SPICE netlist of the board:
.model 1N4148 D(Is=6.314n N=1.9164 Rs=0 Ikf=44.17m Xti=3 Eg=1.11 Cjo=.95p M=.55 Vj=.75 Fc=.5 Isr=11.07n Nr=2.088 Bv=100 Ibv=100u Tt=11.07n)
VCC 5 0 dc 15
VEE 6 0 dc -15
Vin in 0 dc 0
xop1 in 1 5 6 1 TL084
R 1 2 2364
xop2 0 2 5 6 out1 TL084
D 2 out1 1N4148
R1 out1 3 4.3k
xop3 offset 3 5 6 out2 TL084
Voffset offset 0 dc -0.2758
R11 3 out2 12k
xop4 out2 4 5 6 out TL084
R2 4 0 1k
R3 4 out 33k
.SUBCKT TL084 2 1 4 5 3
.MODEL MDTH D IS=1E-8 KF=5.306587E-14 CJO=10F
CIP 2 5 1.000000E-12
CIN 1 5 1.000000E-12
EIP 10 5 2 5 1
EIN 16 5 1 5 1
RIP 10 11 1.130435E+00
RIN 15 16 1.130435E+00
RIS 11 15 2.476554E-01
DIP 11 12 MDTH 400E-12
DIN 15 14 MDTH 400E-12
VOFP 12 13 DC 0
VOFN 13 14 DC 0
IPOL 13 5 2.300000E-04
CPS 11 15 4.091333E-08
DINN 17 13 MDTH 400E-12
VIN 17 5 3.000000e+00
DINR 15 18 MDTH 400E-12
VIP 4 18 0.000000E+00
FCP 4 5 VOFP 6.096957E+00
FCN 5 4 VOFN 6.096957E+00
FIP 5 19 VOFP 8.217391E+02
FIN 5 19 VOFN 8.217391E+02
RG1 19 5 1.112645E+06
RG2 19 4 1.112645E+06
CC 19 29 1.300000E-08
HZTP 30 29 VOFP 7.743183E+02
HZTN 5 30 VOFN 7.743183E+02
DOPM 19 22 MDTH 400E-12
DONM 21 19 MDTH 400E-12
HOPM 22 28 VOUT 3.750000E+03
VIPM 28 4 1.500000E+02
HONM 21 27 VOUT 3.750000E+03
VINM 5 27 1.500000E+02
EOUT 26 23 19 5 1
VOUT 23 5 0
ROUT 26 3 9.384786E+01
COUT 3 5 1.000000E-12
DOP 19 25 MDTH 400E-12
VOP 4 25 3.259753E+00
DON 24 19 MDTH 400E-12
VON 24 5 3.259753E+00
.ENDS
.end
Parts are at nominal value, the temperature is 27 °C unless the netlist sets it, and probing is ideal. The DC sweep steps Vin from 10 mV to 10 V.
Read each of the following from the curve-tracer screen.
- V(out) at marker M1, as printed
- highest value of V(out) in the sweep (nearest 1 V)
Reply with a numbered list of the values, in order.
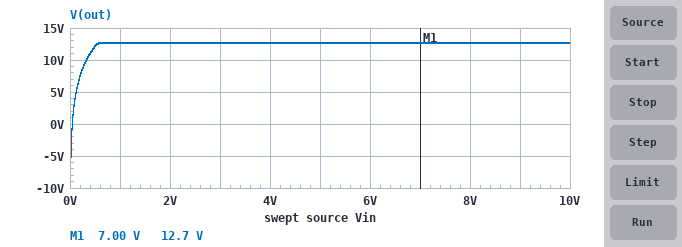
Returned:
1. 12.7 V
2. 13 V
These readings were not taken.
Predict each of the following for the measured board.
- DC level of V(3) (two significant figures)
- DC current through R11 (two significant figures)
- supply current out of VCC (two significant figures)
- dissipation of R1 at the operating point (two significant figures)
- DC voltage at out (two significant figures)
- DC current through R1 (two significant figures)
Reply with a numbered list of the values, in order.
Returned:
1. -280 mV
2. 64 µA
3. 5.7 mA
4. 18 µW
5. -13 V
6. 64 µA
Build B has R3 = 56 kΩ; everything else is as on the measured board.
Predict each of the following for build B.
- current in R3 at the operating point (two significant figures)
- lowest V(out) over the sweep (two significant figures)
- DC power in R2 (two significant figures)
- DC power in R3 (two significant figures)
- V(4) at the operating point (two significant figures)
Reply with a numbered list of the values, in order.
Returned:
1. 220 µA
2. -13 V
3. 50 µW
4. 2.8 mW
5. -220 mV
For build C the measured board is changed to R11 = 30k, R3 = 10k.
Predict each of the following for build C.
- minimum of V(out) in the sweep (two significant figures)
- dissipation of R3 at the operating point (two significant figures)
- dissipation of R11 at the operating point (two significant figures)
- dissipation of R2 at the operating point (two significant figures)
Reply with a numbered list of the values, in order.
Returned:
1. -1.7 V
2. 13 mW
3. 120 µW
4. 1.3 mW
